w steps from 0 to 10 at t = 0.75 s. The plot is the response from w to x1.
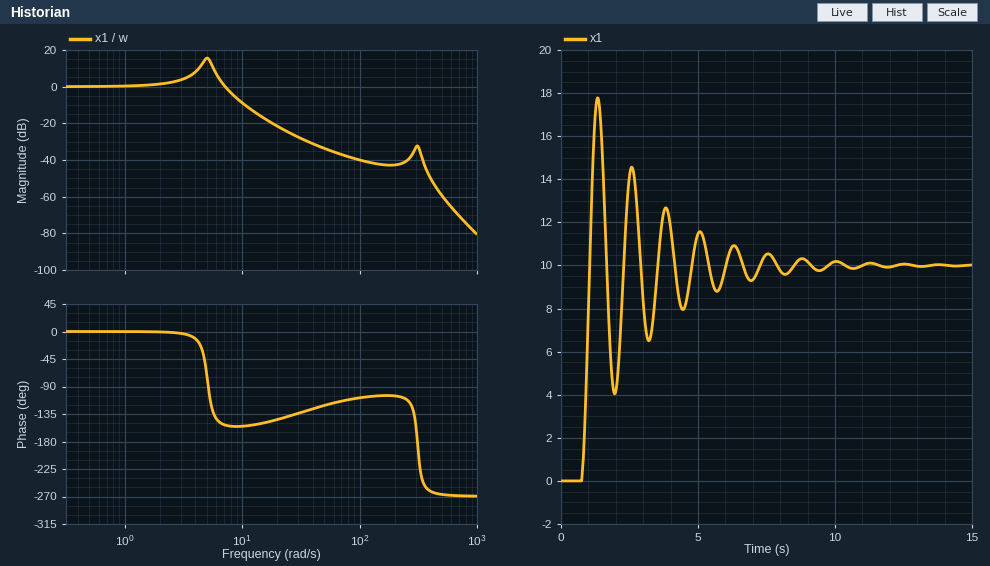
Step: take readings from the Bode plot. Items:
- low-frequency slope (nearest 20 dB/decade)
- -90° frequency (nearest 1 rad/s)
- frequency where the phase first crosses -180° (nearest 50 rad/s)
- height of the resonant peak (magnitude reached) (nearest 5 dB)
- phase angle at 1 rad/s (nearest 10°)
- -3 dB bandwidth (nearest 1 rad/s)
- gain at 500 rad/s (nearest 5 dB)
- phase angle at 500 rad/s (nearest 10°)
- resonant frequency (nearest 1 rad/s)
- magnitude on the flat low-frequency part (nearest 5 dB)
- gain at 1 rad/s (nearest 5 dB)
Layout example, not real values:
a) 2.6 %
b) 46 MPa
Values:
a) 0 dB/decade
b) 5 rad/s
c) 300 rad/s
d) 15 dB
e) 0°
f) 8 rad/s
g) -60 dB
h) -270°
i) 5 rad/s
j) 0 dB
k) 0 dB
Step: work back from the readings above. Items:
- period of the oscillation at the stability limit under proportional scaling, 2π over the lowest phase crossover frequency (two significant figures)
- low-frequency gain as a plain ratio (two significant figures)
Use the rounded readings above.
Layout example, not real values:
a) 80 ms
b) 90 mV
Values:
a) 0.021 s
b) 1.0
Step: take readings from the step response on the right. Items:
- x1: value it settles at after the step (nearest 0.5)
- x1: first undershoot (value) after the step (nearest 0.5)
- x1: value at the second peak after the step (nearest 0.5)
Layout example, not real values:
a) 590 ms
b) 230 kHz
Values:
a) 10.0
b) 4.0
c) 14.5
